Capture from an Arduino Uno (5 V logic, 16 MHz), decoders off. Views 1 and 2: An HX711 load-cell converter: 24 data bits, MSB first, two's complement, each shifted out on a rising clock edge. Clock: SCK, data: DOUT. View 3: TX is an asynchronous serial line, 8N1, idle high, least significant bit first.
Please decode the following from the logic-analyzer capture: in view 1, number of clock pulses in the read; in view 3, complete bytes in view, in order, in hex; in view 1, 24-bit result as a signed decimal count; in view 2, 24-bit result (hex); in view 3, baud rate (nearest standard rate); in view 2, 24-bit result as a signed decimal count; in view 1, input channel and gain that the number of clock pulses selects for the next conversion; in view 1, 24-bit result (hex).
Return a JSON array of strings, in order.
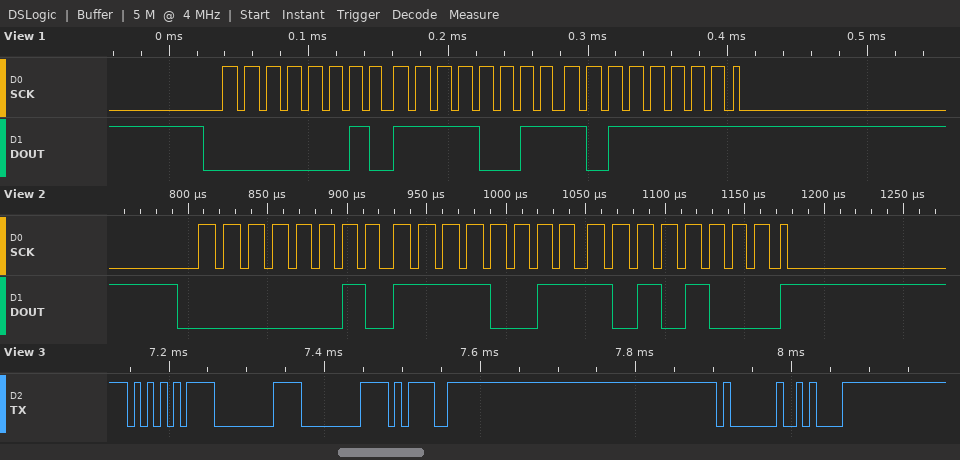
["25", "0x55 0x00 0x00 0x3D 0x01 0x0A", "193471", "0x02F3A8", "115200 baud", "193448", "channel A, gain 128", "0x02F3BF"]
